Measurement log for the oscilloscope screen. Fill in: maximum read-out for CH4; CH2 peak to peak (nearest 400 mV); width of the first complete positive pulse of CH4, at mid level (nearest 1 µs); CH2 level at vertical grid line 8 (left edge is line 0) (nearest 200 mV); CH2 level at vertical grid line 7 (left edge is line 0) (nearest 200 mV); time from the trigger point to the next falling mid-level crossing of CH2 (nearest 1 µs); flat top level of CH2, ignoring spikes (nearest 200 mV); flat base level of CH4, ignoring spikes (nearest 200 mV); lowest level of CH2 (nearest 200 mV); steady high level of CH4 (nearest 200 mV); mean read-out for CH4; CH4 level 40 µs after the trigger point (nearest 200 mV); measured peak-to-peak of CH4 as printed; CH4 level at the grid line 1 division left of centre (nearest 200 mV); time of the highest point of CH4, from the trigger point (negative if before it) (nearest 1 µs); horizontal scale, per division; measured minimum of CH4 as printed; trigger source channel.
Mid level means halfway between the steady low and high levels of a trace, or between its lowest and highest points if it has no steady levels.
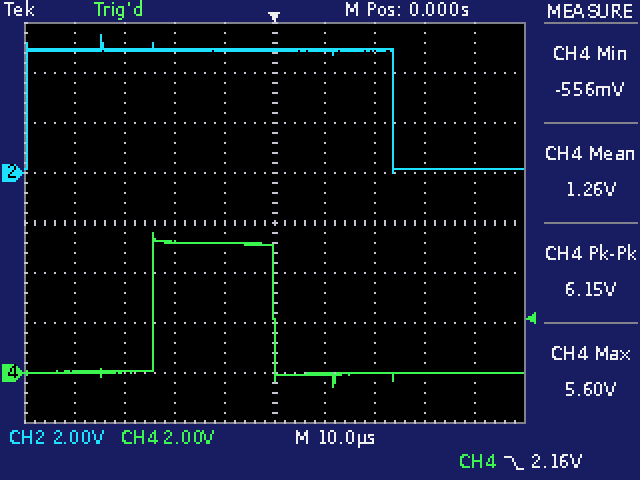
5.60 V
5.6 V
24 µs
200 mV
5.0 V
24 µs
5.0 V
0.0 V
0.0 V
5.2 V
1.26 V
0.0 V
6.15 V
5.2 V
-24 µs
10 µs
-556 mV
CH4
